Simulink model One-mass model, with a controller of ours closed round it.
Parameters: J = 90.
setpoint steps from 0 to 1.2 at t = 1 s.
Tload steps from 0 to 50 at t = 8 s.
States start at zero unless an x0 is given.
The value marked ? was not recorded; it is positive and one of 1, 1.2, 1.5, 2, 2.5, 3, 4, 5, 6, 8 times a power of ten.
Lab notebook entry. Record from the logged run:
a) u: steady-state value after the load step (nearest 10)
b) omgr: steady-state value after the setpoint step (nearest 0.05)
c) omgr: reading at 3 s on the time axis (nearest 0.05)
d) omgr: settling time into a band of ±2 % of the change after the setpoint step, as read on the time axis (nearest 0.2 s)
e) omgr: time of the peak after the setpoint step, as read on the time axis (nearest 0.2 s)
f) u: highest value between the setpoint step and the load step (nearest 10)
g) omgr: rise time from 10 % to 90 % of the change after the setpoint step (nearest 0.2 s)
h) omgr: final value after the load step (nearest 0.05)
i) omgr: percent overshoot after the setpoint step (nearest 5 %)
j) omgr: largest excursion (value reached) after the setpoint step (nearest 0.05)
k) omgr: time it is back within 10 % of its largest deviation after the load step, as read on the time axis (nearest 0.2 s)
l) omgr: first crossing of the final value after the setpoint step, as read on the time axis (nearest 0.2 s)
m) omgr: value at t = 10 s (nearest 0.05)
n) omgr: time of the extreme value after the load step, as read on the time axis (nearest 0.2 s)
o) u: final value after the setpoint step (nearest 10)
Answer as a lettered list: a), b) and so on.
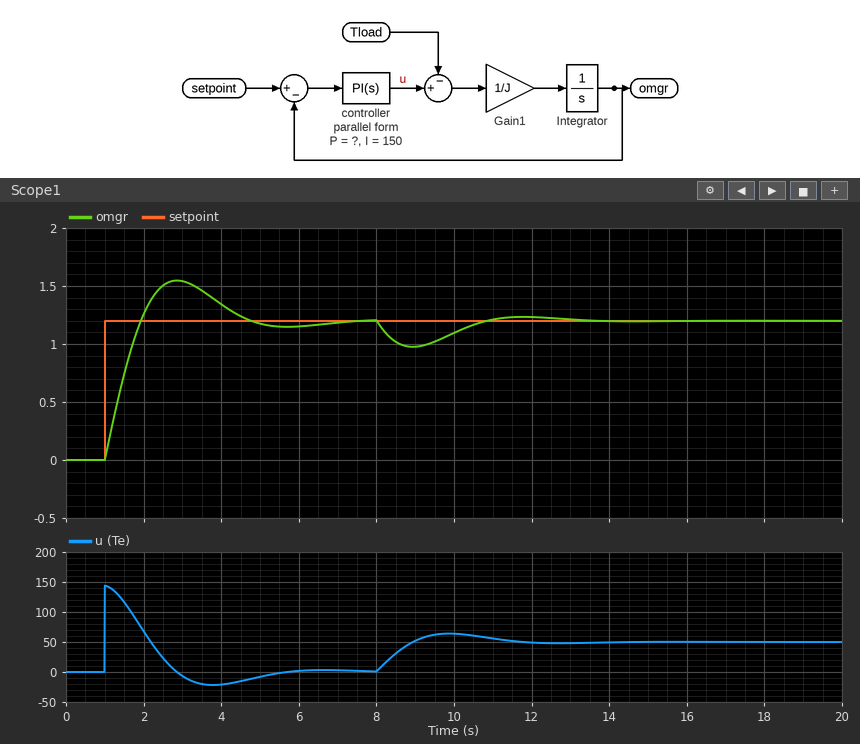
a) 50
b) 1.20
c) 1.55
d) 6.8 s
e) 2.8 s
f) 140
g) 0.8 s
h) 1.20
i) 30 %
j) 1.55
k) 12.6 s
l) 2.0 s
m) 1.10
n) 9.0 s
o) 0
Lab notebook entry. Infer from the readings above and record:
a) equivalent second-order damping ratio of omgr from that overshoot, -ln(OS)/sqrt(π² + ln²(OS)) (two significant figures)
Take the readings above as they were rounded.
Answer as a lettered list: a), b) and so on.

a) 0.36
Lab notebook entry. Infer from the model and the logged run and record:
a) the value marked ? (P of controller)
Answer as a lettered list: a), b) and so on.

a) 120
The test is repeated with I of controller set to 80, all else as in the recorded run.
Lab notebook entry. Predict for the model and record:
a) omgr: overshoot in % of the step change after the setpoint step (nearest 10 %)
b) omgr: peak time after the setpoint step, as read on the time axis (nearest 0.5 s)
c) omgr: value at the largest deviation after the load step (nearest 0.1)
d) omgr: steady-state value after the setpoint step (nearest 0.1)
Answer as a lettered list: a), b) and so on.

a) 20 %
b) 3.5 s
c) 0.9
d) 1.2
